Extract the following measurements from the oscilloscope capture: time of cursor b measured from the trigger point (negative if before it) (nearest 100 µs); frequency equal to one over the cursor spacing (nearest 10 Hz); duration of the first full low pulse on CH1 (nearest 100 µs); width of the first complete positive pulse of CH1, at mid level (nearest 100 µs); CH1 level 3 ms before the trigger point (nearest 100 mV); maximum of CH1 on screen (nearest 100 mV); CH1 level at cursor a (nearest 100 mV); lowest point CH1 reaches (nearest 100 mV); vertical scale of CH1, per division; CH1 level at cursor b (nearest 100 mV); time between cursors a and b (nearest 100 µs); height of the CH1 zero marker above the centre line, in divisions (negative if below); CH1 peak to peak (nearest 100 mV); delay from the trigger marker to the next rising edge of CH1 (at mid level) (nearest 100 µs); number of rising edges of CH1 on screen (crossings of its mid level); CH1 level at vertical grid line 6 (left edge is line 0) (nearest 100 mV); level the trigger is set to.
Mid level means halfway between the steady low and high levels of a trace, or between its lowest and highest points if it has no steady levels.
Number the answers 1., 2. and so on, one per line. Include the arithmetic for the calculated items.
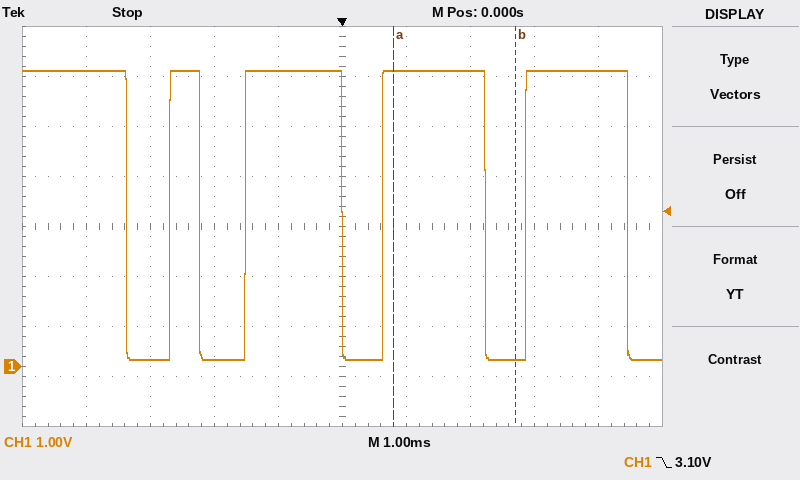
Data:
1. +2.7 ms
2. 1 / 1.9 ms ≈ 530 Hz
3. 700 µs
4. 500 µs
5. 100 mV
6. 5.9 V
7. 5.9 V
8. 100 mV
9. 1 V
10. 100 mV
11. 1.9 ms
12. -2.8 div
13. 5.9 V − (100 mV) = 5.8 V
14. 600 µs
15. 4
16. 5.9 V
17. 3.10 V
